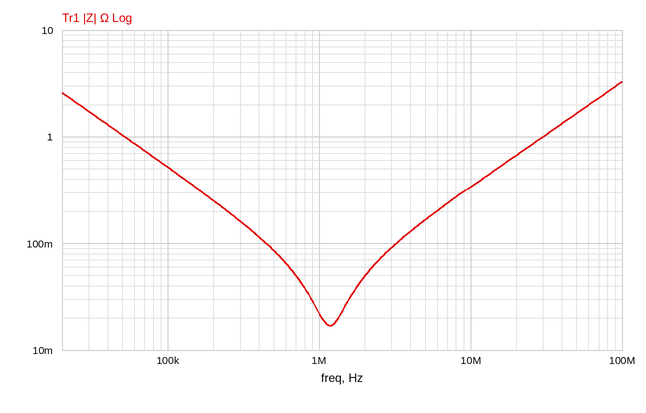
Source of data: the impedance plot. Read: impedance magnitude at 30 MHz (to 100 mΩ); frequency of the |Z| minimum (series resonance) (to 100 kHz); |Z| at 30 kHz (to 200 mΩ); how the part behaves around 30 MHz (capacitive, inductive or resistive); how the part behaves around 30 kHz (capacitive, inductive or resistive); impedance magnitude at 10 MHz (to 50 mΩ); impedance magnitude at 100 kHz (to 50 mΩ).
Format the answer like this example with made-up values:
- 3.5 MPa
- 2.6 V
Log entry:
- 1.0 Ω
- 1.2 MHz
- 1.8 Ω
- inductive
- capacitive
- 350 mΩ
- 500 mΩ
